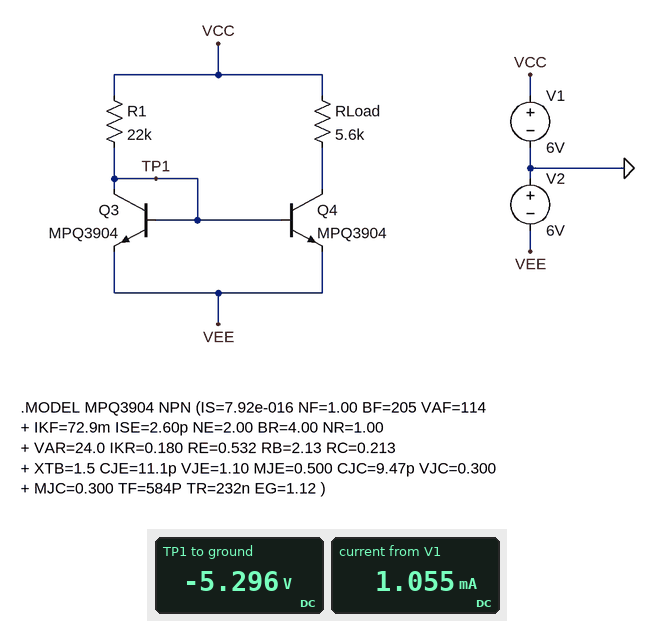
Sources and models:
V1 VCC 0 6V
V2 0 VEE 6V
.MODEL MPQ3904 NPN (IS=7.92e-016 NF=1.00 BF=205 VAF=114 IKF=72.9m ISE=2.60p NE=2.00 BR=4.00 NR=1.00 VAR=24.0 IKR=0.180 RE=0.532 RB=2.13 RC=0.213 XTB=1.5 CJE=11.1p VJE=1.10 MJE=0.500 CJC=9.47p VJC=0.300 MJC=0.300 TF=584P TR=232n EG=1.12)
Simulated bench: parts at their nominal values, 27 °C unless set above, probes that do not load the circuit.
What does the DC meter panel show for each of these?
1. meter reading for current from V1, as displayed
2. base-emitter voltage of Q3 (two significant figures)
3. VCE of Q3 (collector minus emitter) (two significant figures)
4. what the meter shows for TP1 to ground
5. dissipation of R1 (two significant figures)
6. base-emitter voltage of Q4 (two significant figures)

1.055 mA
700 mV
700 mV
-5.296 V
5.8 mW
700 mV
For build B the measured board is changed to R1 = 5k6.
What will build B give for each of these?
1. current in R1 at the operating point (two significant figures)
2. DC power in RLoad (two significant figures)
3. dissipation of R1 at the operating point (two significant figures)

2.0 mA
22 mW
23 mW
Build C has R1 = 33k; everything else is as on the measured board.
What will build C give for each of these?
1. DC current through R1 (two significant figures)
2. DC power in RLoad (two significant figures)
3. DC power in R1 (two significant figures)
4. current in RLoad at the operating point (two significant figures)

340 µA
740 µW
3.9 mW
360 µA
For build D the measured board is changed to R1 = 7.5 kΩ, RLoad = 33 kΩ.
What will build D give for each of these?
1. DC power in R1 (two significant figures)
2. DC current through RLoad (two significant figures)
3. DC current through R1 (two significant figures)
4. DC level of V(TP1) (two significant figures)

17 mW
360 µA
1.5 mA
-5.3 V
